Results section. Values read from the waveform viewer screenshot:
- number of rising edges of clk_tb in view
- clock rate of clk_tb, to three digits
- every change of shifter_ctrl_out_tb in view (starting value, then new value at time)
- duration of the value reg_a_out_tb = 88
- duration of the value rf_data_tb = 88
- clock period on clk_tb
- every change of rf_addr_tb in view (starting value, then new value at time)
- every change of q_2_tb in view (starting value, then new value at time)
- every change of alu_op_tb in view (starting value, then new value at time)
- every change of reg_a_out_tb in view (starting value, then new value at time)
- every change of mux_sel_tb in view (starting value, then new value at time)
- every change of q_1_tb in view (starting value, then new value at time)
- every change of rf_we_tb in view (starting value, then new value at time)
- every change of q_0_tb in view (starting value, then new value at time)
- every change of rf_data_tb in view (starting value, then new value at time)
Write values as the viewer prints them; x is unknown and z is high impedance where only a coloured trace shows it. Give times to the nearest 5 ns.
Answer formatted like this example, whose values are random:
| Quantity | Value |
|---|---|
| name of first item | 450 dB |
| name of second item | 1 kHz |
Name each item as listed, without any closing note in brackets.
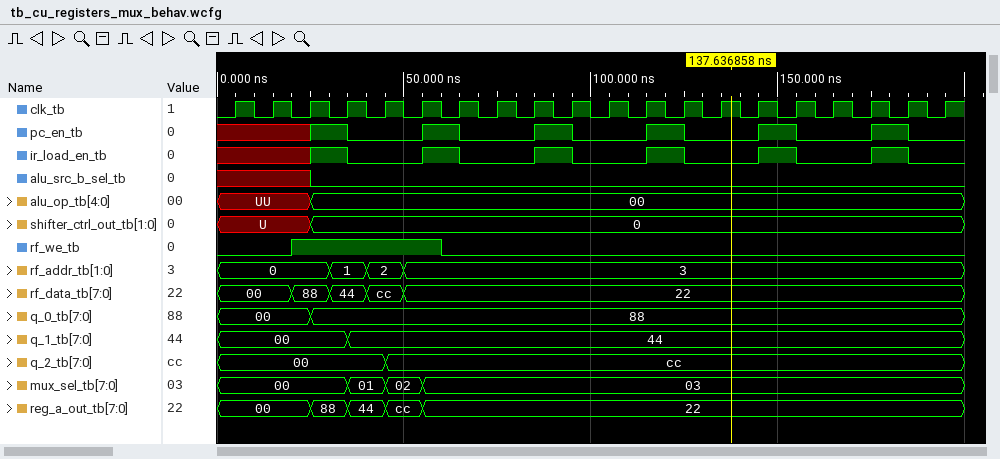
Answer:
| Quantity | Value |
|---|---|
| number of rising edges of clk_tb in view | 20 |
| clock rate of clk_tb, to three digits | 100 MHz |
| every change of shifter_ctrl_out_tb in view | U, 0 at 25 ns |
| duration of the value reg_a_out_tb = 88 | 10 ns |
| duration of the value rf_data_tb = 88 | 10 ns |
| clock period on clk_tb | 10 ns |
| every change of rf_addr_tb in view | 0, 1 at 30 ns, 2 at 40 ns, 3 at 50 ns |
| every change of q_2_tb in view | 00, cc at 45 ns |
| every change of alu_op_tb in view | UU, 00 at 25 ns |
| every change of reg_a_out_tb in view | 00, 88 at 25 ns, 44 at 35 ns, cc at 45 ns, 22 at 55 ns |
| every change of mux_sel_tb in view | 00, 01 at 35 ns, 02 at 45 ns, 03 at 55 ns |
| every change of q_1_tb in view | 00, 44 at 35 ns |
| every change of rf_we_tb in view | 0, 1 at 20 ns, 0 at 60 ns |
| every change of q_0_tb in view | 00, 88 at 25 ns |
| every change of rf_data_tb in view | 00, 88 at 20 ns, 44 at 30 ns, cc at 40 ns, 22 at 50 ns |
